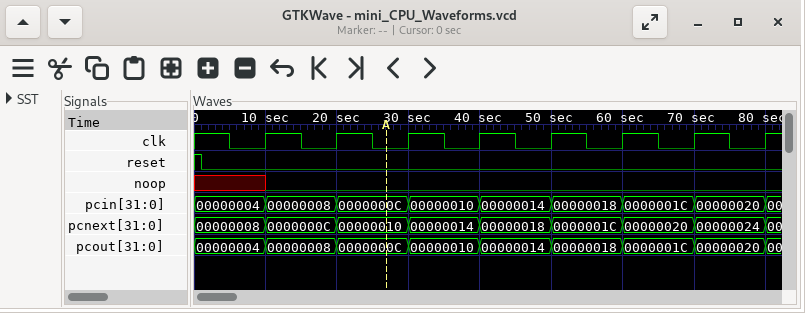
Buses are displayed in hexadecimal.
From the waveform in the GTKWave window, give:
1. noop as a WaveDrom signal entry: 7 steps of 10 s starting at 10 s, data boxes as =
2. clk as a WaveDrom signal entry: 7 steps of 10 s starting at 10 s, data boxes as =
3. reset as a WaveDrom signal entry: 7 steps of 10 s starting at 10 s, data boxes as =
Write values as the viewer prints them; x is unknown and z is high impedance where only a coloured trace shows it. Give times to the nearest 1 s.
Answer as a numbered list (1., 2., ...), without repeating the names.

1. {name: 'noop', wave: '0......'}
2. {name: 'clk', wave: 'p......'}
3. {name: 'reset', wave: '0......'}
